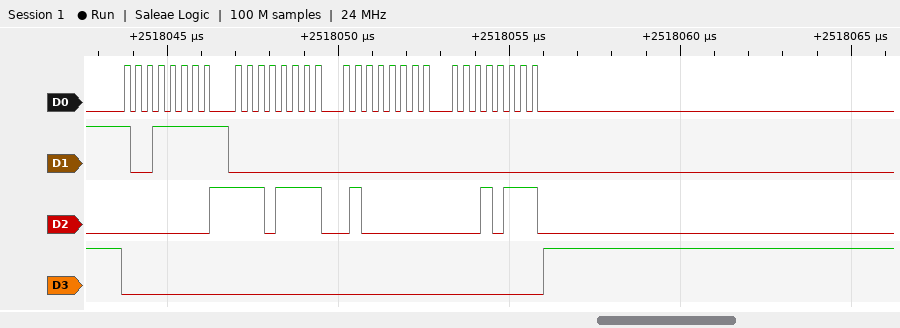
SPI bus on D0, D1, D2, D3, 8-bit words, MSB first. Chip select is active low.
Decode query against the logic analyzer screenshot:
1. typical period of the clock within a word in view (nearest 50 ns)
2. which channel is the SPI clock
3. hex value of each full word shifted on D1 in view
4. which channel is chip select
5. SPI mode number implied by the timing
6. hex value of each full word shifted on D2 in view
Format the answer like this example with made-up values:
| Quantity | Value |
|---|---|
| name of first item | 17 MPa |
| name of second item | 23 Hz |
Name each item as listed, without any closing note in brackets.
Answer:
| Quantity | Value |
|---|---|
| typical period of the clock within a word in view | 350 ns |
| which channel is the SPI clock | D0 |
| hex value of each full word shifted on D1 in view | 9F, 00, 00, 00 |
| which channel is chip select | D3 |
| SPI mode number implied by the timing | 0 |
| hex value of each full word shifted on D2 in view | 00, EF, 40, 17 |
